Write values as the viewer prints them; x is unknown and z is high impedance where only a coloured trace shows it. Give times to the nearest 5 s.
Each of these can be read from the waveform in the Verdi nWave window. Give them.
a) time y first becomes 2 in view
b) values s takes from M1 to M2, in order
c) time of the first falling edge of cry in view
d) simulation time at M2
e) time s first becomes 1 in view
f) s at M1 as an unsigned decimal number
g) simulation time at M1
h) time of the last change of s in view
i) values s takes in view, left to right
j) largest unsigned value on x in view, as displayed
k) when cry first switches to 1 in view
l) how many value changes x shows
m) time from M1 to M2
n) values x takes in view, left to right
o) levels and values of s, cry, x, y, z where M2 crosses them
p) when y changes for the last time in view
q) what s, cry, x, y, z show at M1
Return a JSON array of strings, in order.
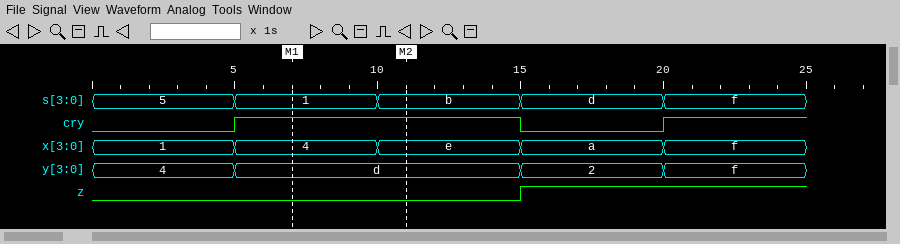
["15 s", "1, b", "15 s", "10 s", "5 s", "1", "5 s", "20 s", "5, 1, b, d, f", "f", "5 s", "4", "5 s", "1, 4, e, a, f", "s=b, cry=1, x=e, y=d, z=0", "20 s", "s=1, cry=1, x=4, y=d, z=0"]
